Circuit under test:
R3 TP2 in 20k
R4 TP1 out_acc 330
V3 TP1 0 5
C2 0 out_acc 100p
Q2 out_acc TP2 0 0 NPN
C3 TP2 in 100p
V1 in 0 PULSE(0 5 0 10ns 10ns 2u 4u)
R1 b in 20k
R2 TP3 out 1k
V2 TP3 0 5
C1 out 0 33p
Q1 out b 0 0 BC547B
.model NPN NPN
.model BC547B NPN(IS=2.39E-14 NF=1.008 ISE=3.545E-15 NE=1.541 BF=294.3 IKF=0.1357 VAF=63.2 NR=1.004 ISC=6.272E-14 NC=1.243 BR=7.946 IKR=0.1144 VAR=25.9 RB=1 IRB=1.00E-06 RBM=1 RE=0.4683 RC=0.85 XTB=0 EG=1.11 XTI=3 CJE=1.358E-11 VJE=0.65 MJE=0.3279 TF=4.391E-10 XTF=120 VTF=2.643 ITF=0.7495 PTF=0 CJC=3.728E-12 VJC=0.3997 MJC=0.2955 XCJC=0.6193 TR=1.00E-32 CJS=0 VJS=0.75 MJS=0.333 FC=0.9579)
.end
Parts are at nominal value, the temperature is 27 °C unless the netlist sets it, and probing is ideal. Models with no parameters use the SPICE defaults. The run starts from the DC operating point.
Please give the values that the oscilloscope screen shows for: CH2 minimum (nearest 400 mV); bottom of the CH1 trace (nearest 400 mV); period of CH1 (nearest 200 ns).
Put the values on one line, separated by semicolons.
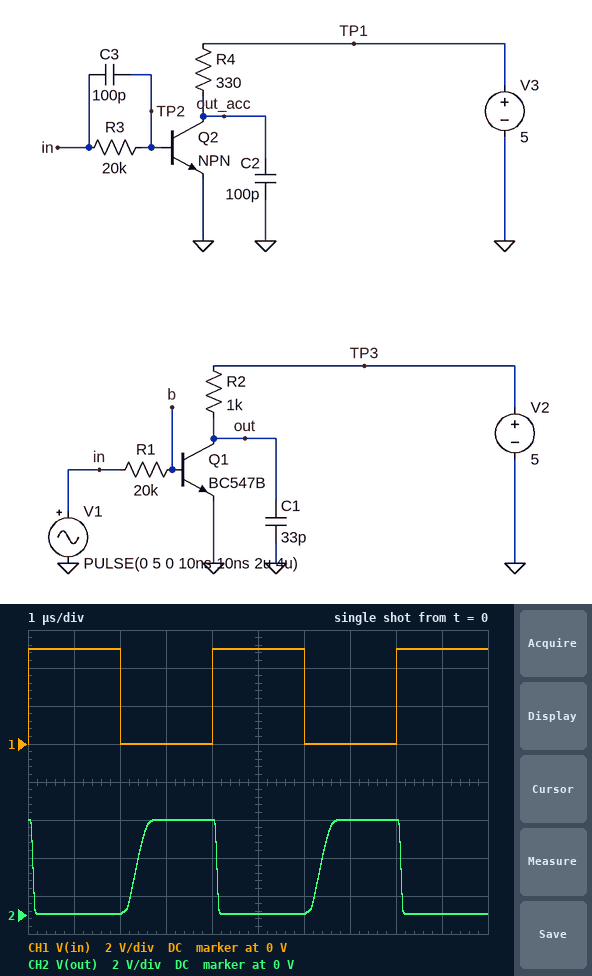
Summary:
0 V; 0 V; 4.0 µs
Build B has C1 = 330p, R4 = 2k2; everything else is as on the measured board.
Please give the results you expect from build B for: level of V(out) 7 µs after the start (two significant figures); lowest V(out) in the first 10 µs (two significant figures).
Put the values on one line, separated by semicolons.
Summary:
4.5 V; 47 mV
